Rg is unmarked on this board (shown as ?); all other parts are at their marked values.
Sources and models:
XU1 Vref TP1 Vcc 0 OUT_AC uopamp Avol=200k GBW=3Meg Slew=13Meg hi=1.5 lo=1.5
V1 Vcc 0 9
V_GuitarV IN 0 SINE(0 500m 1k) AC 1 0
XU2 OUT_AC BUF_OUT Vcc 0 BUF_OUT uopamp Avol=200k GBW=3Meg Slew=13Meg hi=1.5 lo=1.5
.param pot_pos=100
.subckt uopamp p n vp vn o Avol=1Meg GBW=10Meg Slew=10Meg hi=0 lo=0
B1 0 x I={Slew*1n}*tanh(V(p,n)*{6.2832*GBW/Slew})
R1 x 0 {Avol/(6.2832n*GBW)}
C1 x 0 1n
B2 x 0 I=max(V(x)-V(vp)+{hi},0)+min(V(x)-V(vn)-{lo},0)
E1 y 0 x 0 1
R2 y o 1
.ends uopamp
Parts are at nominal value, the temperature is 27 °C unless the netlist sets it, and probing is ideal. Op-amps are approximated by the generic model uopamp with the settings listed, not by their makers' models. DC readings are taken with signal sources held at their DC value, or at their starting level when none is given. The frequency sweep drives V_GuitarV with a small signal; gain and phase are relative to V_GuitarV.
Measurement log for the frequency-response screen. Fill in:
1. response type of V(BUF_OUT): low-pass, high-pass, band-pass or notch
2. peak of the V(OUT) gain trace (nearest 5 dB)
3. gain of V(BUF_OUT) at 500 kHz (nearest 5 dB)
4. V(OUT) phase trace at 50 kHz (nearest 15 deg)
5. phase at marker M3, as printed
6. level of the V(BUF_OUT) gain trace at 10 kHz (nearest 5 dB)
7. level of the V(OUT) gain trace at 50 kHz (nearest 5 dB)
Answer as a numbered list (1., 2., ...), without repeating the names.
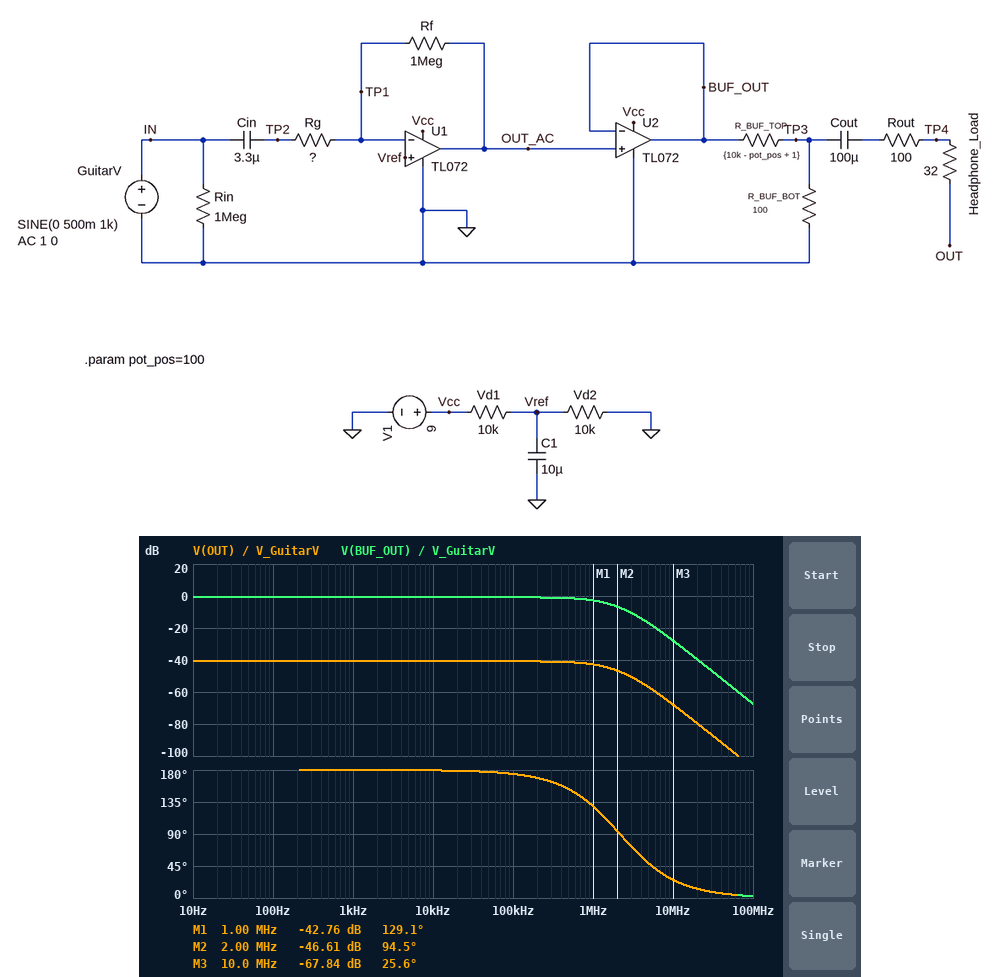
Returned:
1. low-pass
2. -40 dB
3. 0 dB
4. 180 deg
5. 25.6 deg
6. 0 dB
7. -40 dB
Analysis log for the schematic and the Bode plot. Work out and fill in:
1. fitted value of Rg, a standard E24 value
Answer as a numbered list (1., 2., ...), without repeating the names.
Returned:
1. 1.1 MΩ
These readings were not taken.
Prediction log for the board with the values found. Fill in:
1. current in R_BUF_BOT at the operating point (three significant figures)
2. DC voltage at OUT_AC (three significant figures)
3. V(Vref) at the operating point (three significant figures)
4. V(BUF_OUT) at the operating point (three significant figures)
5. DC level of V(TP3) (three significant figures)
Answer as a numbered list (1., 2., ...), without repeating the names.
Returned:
1. 450 µA
2. 4.50 V
3. 4.50 V
4. 4.50 V
5. 45.0 mV
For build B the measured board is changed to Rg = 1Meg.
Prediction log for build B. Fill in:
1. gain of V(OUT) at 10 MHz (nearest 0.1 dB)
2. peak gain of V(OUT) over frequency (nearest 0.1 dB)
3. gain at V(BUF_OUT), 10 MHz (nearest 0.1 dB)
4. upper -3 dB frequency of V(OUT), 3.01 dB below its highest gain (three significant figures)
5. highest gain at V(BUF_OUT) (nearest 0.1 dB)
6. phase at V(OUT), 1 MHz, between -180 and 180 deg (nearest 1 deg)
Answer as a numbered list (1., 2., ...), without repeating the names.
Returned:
1. -67.4 dB
2. -40.0 dB
3. -27.4 dB
4. 1.26 MHz
5. 0 dB
6. 128 deg
